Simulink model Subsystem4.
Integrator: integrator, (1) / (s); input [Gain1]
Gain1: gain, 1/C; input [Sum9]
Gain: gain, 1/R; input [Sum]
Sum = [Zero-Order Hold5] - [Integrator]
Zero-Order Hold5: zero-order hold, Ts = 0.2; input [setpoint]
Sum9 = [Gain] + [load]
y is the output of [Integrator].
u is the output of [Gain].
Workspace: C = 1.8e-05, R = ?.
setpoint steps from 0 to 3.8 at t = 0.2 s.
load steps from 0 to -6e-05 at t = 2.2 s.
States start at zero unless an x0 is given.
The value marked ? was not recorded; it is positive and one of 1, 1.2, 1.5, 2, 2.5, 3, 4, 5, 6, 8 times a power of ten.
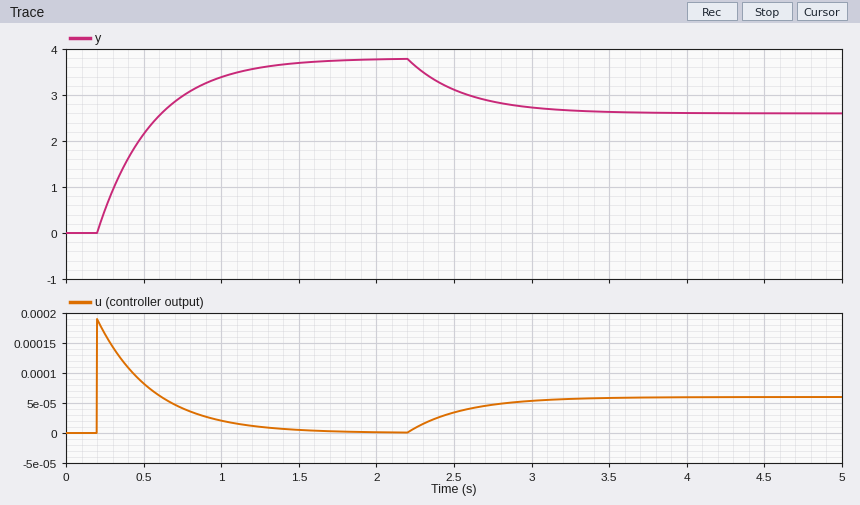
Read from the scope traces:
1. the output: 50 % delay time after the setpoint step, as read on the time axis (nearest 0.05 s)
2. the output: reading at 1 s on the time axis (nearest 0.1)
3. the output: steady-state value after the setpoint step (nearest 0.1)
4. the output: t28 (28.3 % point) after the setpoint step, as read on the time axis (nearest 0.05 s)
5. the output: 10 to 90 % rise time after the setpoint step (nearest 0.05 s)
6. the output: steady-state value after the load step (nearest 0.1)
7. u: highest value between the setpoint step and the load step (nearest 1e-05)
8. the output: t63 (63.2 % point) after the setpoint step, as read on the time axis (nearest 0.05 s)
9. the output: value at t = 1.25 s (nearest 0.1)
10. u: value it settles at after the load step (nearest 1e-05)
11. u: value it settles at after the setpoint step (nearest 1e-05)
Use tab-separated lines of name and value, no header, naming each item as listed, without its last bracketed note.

the output: 50 % delay time after the setpoint step, as read on the time axis	0.45 s
the output: reading at 1 s on the time axis	3.4
the output: steady-state value after the setpoint step	3.8
the output: t28 (28.3 % point) after the setpoint step, as read on the time axis	0.30 s
the output: 10 to 90 % rise time after the setpoint step	0.80 s
the output: steady-state value after the load step	2.6
u: highest value between the setpoint step and the load step	0.00019
the output: t63 (63.2 % point) after the setpoint step, as read on the time axis	0.55 s
the output: value at t = 1.25 s	3.6
u: value it settles at after the load step	0.00006
u: value it settles at after the setpoint step	0.00000
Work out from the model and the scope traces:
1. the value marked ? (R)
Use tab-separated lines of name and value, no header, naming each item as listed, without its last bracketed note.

the value marked ?	20000
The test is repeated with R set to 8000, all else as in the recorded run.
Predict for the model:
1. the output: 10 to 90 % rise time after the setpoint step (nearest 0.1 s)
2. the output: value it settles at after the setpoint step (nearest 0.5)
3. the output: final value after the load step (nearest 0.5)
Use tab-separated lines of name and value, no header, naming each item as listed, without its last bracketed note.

the output: 10 to 90 % rise time after the setpoint step	0.3 s
the output: value it settles at after the setpoint step	4.0
the output: final value after the load step	3.5
